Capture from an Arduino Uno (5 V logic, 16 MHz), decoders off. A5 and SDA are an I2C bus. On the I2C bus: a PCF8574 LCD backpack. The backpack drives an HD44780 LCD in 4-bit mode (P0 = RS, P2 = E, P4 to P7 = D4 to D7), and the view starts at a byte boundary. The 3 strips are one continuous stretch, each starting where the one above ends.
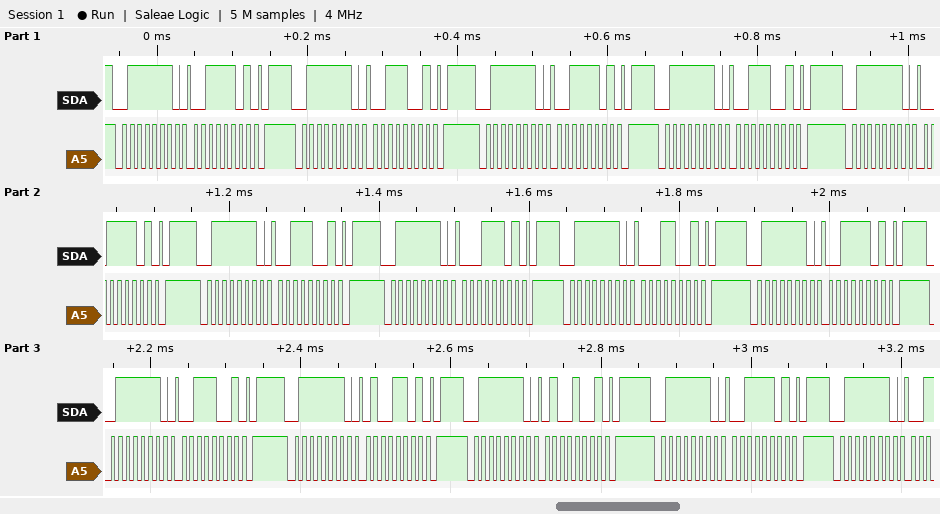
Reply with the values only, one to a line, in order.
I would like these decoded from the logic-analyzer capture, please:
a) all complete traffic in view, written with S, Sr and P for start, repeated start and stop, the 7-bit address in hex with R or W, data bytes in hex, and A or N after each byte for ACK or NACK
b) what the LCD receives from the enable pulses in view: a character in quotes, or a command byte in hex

S 3FW A 3D A P S 3FW A 39 A P S 3FW A 3D A P S 3FW A 39 A P S 3FW A 3D A P S 3FW A 39 A P S 3FW A 1D A P S 3FW A 19 A P S 3FW A 3D A P S 3FW A 39 A P S 3FW A 4D A P S 3FW A 49 A P S 3FW A 3D A P S 3FW A
'3' '1' '4'
